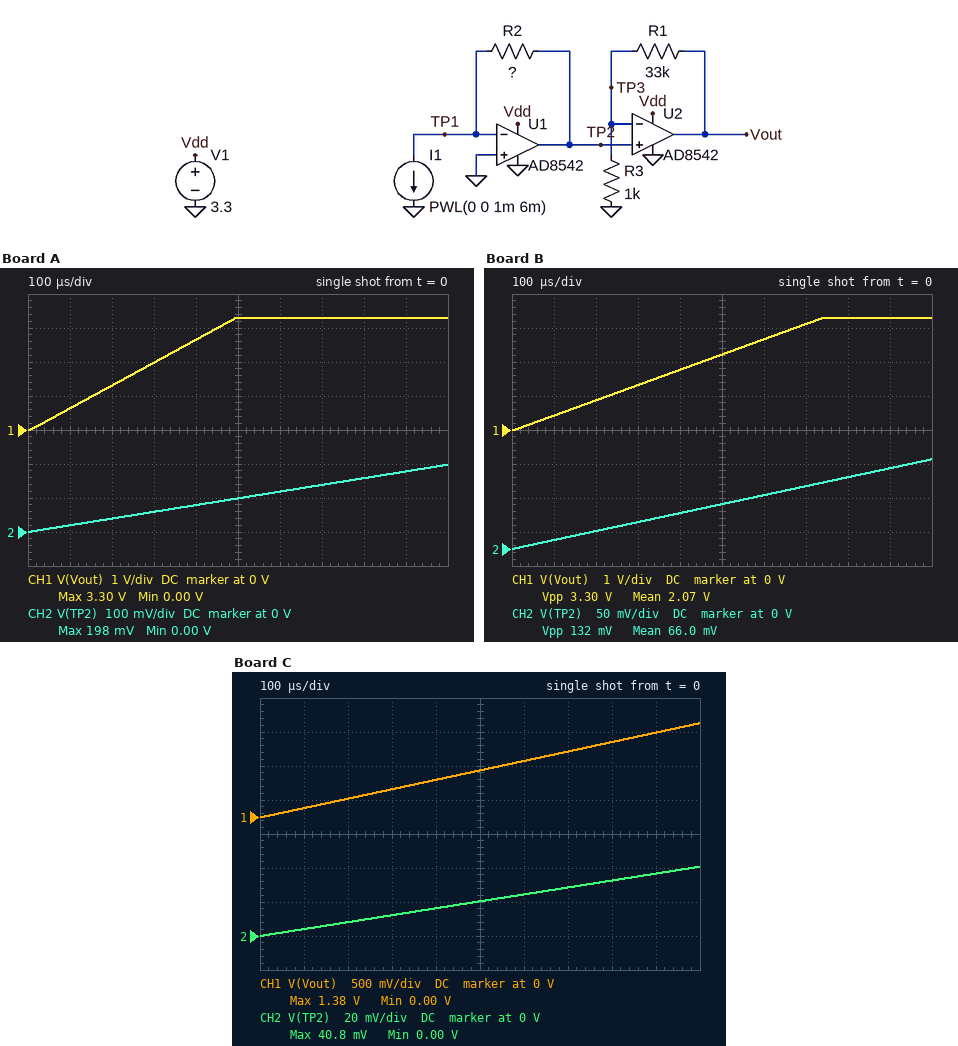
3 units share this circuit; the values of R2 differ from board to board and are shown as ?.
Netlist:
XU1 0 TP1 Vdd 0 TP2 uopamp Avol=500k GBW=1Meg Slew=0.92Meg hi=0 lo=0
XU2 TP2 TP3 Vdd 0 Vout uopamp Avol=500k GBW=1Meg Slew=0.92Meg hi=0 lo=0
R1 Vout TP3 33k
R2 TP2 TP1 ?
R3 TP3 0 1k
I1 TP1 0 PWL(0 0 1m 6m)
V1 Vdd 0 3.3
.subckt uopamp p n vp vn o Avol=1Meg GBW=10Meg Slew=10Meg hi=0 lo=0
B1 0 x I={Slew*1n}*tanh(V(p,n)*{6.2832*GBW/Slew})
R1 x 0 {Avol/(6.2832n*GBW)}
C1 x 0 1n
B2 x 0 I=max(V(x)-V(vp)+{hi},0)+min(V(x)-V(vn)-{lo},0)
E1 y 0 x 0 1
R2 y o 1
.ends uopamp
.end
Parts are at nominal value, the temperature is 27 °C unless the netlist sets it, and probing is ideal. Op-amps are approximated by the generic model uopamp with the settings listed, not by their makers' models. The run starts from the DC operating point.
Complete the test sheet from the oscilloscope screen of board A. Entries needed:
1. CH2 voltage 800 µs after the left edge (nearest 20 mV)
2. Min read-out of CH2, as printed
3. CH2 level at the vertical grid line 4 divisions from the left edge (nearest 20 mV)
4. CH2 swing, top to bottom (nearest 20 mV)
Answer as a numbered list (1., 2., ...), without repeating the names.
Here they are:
1. 160 mV
2. 0.00 V
3. 80 mV
4. 200 mV
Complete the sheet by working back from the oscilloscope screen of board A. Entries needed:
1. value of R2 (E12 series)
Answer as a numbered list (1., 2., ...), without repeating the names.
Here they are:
1. 33 Ω
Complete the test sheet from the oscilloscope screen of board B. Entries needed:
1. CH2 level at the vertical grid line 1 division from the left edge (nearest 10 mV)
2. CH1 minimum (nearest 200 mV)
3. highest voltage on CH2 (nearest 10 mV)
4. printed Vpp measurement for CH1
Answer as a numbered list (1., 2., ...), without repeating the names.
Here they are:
1. 10 mV
2. 0 V
3. 130 mV
4. 3.30 V
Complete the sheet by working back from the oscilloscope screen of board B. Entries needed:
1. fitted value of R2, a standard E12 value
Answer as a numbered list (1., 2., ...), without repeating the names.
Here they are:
1. 22 Ω
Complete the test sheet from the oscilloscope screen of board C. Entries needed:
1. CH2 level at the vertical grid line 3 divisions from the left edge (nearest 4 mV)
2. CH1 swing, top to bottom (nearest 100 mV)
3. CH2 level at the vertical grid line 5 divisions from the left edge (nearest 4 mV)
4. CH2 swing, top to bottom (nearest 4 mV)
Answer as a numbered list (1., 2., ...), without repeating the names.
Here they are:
1. 12 mV
2. 1.4 V
3. 20 mV
4. 40 mV
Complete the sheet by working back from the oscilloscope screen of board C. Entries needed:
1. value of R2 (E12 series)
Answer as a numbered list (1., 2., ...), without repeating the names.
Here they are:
1. 6.8 Ω
